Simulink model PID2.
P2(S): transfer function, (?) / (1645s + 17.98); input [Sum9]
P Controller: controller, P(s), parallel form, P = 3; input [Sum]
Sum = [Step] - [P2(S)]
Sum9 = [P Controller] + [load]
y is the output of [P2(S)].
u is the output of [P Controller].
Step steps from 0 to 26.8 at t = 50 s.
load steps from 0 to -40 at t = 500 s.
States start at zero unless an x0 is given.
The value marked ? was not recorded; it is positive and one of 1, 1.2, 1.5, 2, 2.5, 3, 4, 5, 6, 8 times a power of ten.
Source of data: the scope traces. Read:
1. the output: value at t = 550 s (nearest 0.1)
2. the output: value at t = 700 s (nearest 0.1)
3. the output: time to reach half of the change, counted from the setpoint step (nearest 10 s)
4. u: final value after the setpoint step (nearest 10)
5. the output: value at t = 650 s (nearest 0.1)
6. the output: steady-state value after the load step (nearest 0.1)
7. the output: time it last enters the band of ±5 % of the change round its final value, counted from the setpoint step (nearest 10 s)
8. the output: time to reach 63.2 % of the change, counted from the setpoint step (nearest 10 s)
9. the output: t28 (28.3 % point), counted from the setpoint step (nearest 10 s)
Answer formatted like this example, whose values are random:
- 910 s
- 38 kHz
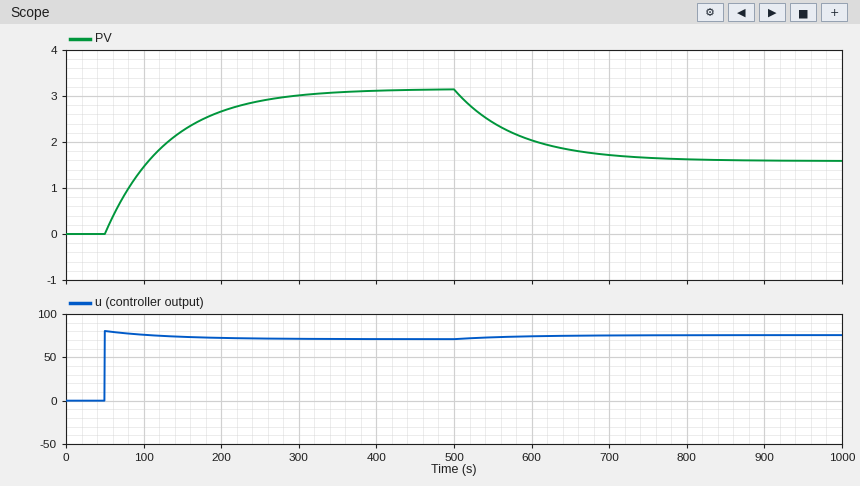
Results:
- 2.4
- 1.7
- 60 s
- 70
- 1.8
- 1.6
- 240 s
- 80 s
- 30 s
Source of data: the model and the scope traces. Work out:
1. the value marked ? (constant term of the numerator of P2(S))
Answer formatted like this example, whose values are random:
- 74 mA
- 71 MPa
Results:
- 0.8
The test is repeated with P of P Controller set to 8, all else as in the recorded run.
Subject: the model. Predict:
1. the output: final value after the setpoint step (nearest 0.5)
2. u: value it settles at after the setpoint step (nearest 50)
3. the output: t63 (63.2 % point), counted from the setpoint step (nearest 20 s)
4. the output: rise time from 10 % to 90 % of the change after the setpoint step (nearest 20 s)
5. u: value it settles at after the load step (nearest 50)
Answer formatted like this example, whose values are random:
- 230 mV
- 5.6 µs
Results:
- 7.0
- 150
- 60 s
- 140 s
- 150
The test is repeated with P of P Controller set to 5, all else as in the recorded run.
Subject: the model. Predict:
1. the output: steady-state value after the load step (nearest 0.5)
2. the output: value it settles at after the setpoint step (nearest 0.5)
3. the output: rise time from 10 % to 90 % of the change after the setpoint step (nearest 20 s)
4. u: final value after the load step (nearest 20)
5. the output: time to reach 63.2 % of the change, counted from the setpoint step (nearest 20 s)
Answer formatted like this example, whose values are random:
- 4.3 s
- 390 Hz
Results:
- 3.5
- 5.0
- 160 s
- 120
- 80 s
